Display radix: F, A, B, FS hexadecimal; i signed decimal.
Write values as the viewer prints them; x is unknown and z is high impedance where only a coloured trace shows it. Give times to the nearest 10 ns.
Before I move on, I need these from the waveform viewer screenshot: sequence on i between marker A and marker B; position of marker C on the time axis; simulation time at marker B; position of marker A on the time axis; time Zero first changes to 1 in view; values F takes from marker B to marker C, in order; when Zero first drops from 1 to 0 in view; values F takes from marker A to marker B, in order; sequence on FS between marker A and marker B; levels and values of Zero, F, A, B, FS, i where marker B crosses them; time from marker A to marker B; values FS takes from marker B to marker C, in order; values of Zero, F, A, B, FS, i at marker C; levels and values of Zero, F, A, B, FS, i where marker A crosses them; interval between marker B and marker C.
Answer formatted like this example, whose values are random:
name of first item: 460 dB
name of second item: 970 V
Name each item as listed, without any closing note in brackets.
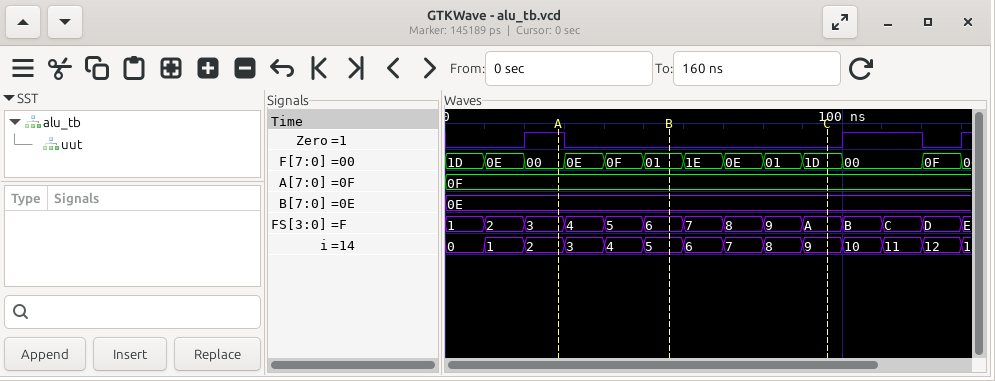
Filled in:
sequence on i between marker A and marker B: 2, 3, 4, 5
position of marker C on the time axis: 100 ns
simulation time at marker B: 60 ns
position of marker A on the time axis: 30 ns
time Zero first changes to 1 in view: 20 ns
values F takes from marker B to marker C, in order: 01, 1E, 0E, 01, 1D
when Zero first drops from 1 to 0 in view: 30 ns
values F takes from marker A to marker B, in order: 00, 0E, 0F, 01
sequence on FS between marker A and marker B: 3, 4, 5, 6
levels and values of Zero, F, A, B, FS, i where marker B crosses them: Zero=0, F=01, A=0F, B=0E, FS=6, i=5
time from marker A to marker B: 30 ns
values FS takes from marker B to marker C, in order: 6, 7, 8, 9, A
values of Zero, F, A, B, FS, i at marker C: Zero=0, F=1D, A=0F, B=0E, FS=A, i=9
levels and values of Zero, F, A, B, FS, i where marker A crosses them: Zero=1, F=00, A=0F, B=0E, FS=3, i=2
interval between marker B and marker C: 40 ns
